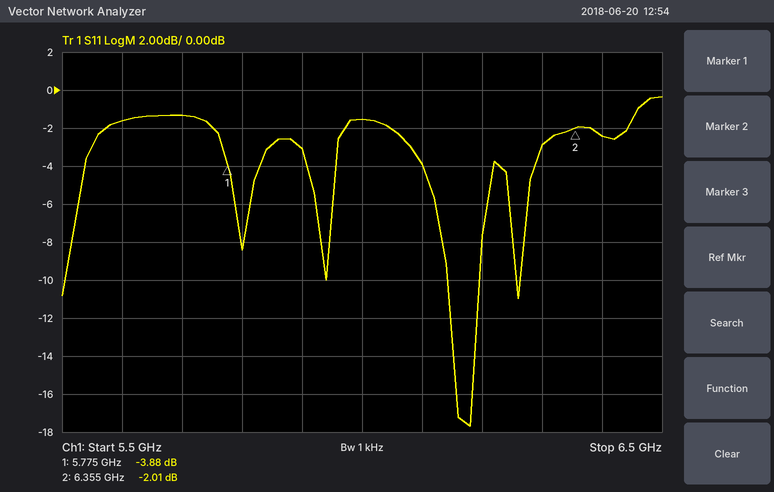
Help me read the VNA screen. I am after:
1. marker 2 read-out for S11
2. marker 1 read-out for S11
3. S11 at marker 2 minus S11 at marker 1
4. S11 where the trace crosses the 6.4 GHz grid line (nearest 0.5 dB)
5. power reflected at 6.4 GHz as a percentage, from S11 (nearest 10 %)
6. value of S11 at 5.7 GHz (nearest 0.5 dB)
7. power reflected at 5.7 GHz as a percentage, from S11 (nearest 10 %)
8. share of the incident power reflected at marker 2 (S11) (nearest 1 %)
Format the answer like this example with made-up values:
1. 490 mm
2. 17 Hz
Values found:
1. -2.01 dB
2. -3.88 dB
3. 1.87 dB
4. -2.5 dB
5. 60 %
6. -1.5 dB
7. 70 %
8. 63 %
